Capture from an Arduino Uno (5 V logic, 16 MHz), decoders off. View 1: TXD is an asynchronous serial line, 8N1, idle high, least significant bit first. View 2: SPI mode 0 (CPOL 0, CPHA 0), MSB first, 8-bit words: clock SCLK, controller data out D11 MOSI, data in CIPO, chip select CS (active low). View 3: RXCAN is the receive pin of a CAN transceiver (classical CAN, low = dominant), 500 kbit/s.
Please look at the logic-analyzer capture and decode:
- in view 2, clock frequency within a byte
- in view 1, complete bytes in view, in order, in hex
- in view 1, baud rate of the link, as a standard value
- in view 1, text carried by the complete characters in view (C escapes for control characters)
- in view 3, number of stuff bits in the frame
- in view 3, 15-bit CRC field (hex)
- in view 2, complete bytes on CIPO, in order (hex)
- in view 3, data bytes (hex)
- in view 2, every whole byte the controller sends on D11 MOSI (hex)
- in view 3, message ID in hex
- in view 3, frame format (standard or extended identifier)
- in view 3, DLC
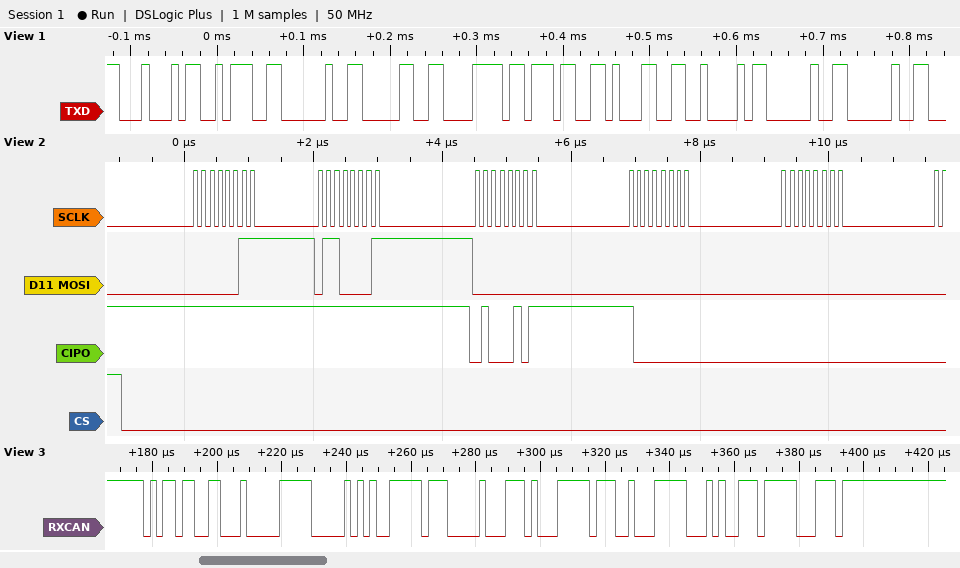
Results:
8 MHz
44 3A 20 30 78 37 31 42 20 20
115200 baud
"D: 0x71B  "
8
0x1DF3
FF FF 45 80 00
3C 14 FF 00 E8 FF 23 E5
03 61 00 00 00
0x5B3
standard
8
